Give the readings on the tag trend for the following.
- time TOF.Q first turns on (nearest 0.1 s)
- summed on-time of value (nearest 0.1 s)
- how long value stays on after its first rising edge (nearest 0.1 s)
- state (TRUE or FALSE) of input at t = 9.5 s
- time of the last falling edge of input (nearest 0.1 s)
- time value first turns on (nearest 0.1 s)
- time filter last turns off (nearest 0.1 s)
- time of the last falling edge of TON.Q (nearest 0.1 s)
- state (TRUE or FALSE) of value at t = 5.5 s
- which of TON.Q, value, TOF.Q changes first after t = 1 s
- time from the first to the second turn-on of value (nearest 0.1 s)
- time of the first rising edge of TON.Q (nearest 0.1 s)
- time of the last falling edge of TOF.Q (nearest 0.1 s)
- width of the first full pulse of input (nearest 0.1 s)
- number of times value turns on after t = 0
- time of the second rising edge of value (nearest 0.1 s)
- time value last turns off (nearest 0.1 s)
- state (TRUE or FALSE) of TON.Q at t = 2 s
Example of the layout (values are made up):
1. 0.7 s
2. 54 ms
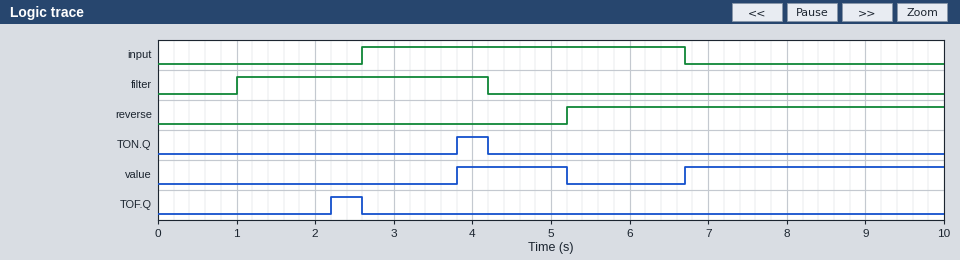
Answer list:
1. 2.2 s
2. 4.7 s
3. 1.4 s
4. FALSE
5. 6.7 s
6. 3.8 s
7. 4.2 s
8. 4.2 s
9. FALSE
10. TOF.Q
11. 2.9 s
12. 3.8 s
13. 2.6 s
14. 4.1 s
15. 2
16. 6.7 s
17. 5.2 s
18. FALSE
